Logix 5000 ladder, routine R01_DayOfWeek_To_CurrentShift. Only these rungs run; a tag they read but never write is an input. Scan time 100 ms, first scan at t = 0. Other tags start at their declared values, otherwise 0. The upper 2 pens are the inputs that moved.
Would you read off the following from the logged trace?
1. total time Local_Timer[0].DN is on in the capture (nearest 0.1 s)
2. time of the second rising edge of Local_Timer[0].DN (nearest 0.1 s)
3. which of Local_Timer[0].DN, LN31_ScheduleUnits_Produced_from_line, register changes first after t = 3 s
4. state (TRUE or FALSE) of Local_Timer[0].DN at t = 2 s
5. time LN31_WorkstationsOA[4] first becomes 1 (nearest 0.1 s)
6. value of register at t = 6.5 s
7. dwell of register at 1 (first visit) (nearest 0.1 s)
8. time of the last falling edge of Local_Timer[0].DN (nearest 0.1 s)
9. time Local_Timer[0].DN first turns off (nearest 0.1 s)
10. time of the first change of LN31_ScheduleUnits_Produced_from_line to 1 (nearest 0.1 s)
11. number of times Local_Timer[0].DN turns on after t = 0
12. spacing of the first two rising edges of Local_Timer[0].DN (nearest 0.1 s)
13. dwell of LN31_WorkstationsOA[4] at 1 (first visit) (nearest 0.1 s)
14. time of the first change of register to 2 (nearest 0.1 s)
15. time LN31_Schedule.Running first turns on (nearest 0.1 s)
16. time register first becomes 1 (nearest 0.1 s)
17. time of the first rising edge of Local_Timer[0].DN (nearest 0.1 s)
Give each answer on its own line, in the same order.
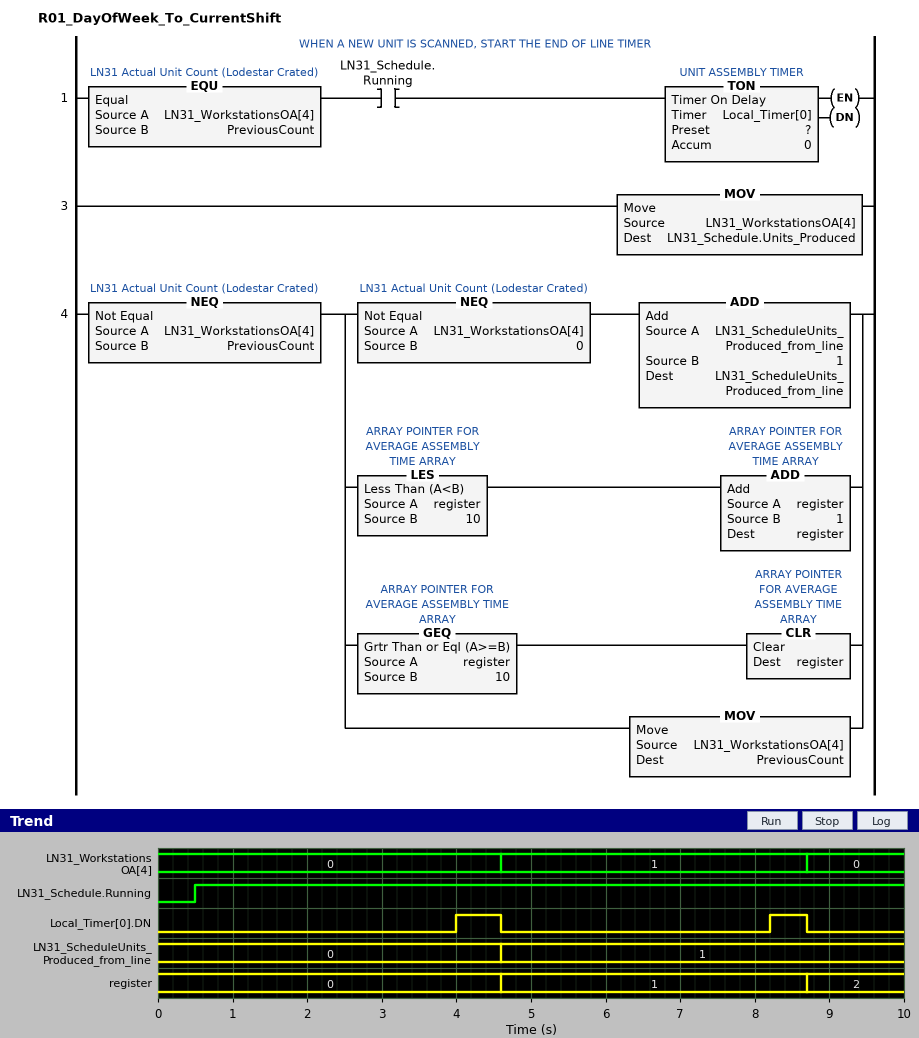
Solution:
1.1 s
8.2 s
Local_Timer[0].DN
FALSE
4.6 s
1
4.1 s
8.7 s
4.6 s
4.6 s
2
4.2 s
4.1 s
8.7 s
0.5 s
4.6 s
4.0 s
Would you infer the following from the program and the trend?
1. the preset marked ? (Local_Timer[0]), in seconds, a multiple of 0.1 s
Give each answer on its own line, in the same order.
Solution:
3.5 s
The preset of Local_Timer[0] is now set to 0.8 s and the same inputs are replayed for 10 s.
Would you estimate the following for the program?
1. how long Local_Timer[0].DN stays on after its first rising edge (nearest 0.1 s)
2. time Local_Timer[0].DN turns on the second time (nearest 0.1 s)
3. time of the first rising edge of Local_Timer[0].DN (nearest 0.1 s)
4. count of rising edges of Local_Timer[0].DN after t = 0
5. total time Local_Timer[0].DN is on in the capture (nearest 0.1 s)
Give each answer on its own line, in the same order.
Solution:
3.3 s
5.5 s
1.3 s
3
6.9 s
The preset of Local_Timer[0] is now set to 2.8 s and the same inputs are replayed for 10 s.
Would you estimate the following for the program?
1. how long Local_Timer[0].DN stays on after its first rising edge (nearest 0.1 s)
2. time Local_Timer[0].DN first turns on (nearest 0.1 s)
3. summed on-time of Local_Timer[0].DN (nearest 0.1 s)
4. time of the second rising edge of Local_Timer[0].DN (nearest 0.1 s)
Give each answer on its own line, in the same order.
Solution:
1.3 s
3.3 s
2.5 s
7.5 s
